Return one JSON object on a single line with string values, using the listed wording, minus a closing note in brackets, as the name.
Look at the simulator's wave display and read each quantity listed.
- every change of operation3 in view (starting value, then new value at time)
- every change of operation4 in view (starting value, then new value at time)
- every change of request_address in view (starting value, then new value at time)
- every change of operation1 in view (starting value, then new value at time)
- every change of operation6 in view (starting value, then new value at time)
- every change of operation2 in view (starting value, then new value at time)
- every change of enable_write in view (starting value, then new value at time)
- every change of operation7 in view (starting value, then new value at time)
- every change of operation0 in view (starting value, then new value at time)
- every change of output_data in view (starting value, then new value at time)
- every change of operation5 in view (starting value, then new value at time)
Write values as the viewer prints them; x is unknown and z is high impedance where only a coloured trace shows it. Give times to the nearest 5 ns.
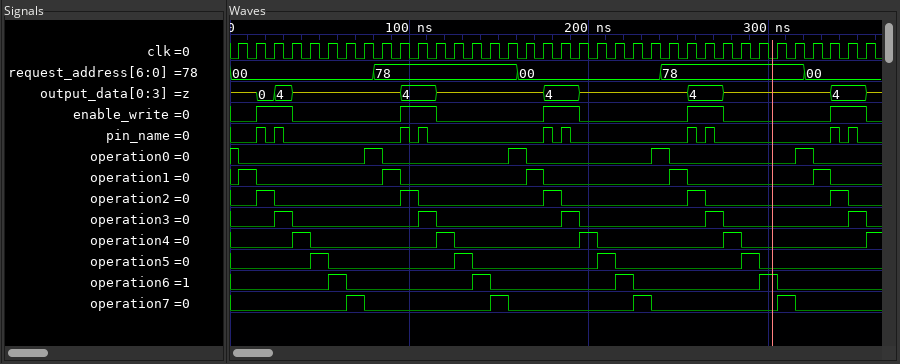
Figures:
{"every change of operation3 in view": "0, 1 at 25 ns, 0 at 35 ns, 1 at 105 ns, 0 at 115 ns, 1 at 185 ns, 0 at 195 ns, 1 at 265 ns, 0 at 275 ns, 1 at 345 ns, 0 at 355 ns", "every change of operation4 in view": "0, 1 at 35 ns, 0 at 45 ns, 1 at 115 ns, 0 at 125 ns, 1 at 195 ns, 0 at 205 ns, 1 at 275 ns, 0 at 285 ns, 1 at 355 ns", "every change of request_address in view": "00, 78 at 80 ns, 00 at 160 ns, 78 at 240 ns, 00 at 320 ns", "every change of operation1 in view": "0, 1 at 5 ns, 0 at 15 ns, 1 at 85 ns, 0 at 95 ns, 1 at 165 ns, 0 at 175 ns, 1 at 245 ns, 0 at 255 ns, 1 at 325 ns, 0 at 335 ns", "every change of operation6 in view": "0, 1 at 55 ns, 0 at 65 ns, 1 at 135 ns, 0 at 145 ns, 1 at 215 ns, 0 at 225 ns, 1 at 295 ns, 0 at 305 ns", "every change of operation2 in view": "0, 1 at 15 ns, 0 at 25 ns, 1 at 95 ns, 0 at 105 ns, 1 at 175 ns, 0 at 185 ns, 1 at 255 ns, 0 at 265 ns, 1 at 335 ns, 0 at 345 ns", "every change of enable_write in view": "0, 1 at 15 ns, 0 at 35 ns, 1 at 95 ns, 0 at 115 ns, 1 at 175 ns, 0 at 195 ns, 1 at 255 ns, 0 at 275 ns, 1 at 335 ns, 0 at 355 ns", "every change of operation7 in view": "0, 1 at 65 ns, 0 at 75 ns, 1 at 145 ns, 0 at 155 ns, 1 at 225 ns, 0 at 235 ns, 1 at 305 ns, 0 at 315 ns", "every change of operation0 in view": "1, 0 at 5 ns, 1 at 75 ns, 0 at 85 ns, 1 at 155 ns, 0 at 165 ns, 1 at 235 ns, 0 at 245 ns, 1 at 315 ns, 0 at 325 ns", "every change of output_data in view": "z, 0 at 15 ns, 4 at 25 ns, z at 35 ns, 4 at 95 ns, z at 115 ns, 4 at 175 ns, z at 195 ns, 4 at 255 ns, z at 275 ns, 4 at 335 ns, z at 355 ns", "every change of operation5 in view": "0, 1 at 45 ns, 0 at 55 ns, 1 at 125 ns, 0 at 135 ns, 1 at 205 ns, 0 at 215 ns, 1 at 285 ns, 0 at 295 ns"}
